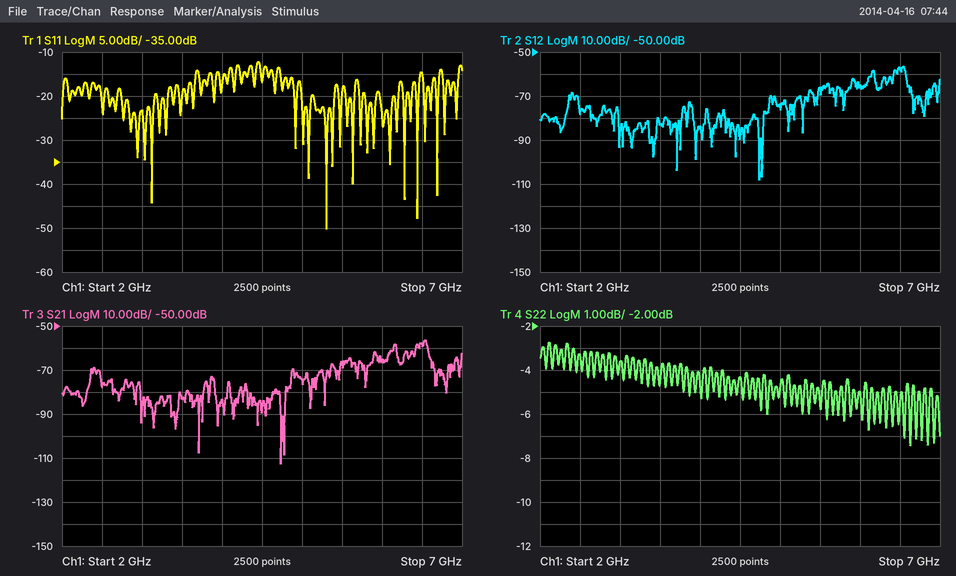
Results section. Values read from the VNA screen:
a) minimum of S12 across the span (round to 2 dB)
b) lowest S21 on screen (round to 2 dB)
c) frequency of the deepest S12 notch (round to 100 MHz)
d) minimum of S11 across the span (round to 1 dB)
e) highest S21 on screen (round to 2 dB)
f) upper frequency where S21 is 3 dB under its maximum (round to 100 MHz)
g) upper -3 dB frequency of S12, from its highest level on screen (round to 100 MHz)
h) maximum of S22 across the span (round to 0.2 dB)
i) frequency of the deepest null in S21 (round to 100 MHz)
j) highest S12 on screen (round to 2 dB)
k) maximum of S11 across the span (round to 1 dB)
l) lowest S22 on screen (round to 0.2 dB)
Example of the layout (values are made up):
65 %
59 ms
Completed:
-108 dB
-112 dB
4.7 GHz
-50 dB
-56 dB
6.6 GHz
6.6 GHz
-2.8 dB
4.7 GHz
-56 dB
-12 dB
-7.4 dB
